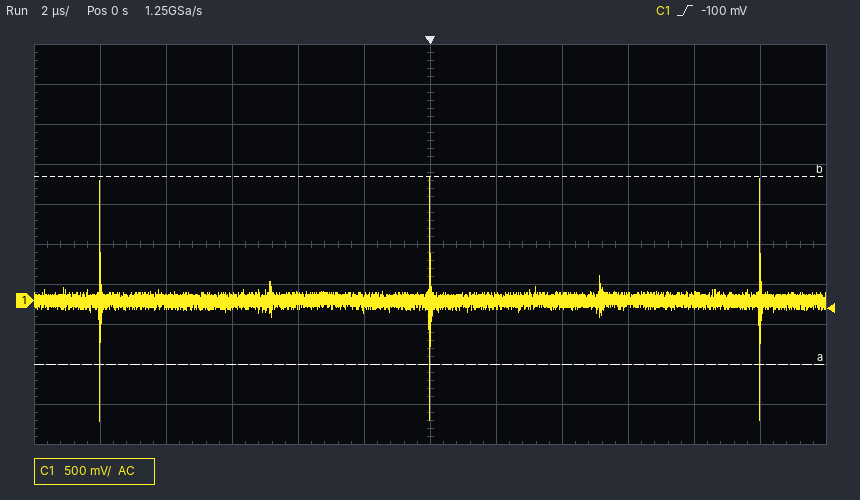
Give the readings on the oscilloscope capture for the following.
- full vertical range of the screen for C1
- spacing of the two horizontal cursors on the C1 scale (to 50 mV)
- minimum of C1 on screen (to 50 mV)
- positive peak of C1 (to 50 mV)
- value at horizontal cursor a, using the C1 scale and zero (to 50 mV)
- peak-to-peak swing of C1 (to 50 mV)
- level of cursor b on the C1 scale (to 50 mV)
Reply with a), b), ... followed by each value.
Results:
a) 5 V
b) 2.35 V
c) -1.50 V
d) 1.55 V
e) -800 mV
f) 3.05 V
g) 1.55 V
